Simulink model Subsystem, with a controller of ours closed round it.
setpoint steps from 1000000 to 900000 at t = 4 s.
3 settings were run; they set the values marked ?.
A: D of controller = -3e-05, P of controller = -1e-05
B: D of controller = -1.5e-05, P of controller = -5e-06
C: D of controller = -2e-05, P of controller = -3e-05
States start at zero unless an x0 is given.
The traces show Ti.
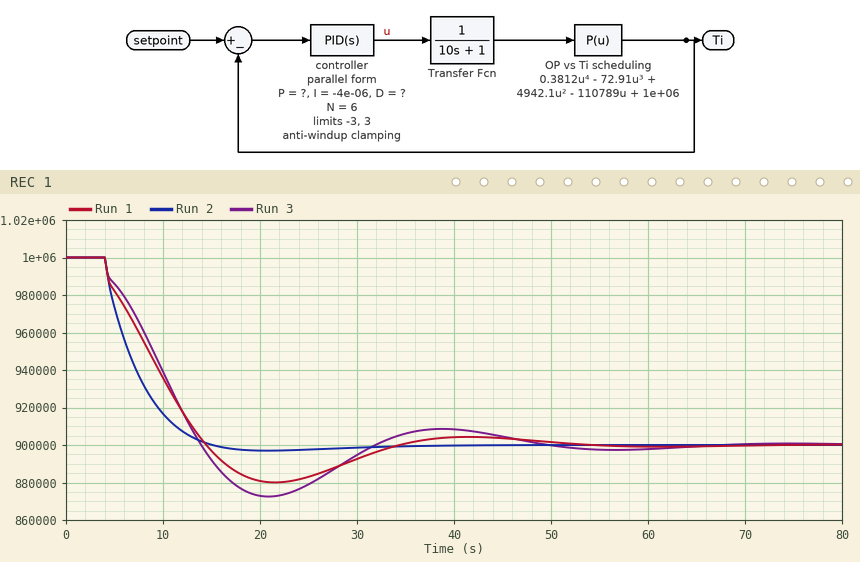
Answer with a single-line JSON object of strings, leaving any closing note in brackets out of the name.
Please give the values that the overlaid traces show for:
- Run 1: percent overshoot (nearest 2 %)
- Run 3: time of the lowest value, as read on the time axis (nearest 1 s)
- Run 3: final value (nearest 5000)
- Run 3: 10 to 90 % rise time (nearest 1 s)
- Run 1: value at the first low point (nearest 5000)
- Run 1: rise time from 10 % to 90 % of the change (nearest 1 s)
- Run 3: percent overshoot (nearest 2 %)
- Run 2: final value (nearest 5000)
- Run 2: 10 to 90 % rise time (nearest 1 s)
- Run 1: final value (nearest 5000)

{"Run 1: percent overshoot": "20 %", "Run 3: time of the lowest value, as read on the time axis": "21 s", "Run 3: final value": "900000", "Run 3: 10 to 90 % rise time": "8 s", "Run 1: value at the first low point": "880000", "Run 1: rise time from 10 % to 90 % of the change": "9 s", "Run 3: percent overshoot": "28 %", "Run 2: final value": "900000", "Run 2: 10 to 90 % rise time": "7 s", "Run 1: final value": "900000"}
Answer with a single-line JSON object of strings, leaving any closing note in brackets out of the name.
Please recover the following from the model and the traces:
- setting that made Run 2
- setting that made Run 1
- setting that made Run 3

{"setting that made Run 2": "C", "setting that made Run 1": "A", "setting that made Run 3": "B"}
